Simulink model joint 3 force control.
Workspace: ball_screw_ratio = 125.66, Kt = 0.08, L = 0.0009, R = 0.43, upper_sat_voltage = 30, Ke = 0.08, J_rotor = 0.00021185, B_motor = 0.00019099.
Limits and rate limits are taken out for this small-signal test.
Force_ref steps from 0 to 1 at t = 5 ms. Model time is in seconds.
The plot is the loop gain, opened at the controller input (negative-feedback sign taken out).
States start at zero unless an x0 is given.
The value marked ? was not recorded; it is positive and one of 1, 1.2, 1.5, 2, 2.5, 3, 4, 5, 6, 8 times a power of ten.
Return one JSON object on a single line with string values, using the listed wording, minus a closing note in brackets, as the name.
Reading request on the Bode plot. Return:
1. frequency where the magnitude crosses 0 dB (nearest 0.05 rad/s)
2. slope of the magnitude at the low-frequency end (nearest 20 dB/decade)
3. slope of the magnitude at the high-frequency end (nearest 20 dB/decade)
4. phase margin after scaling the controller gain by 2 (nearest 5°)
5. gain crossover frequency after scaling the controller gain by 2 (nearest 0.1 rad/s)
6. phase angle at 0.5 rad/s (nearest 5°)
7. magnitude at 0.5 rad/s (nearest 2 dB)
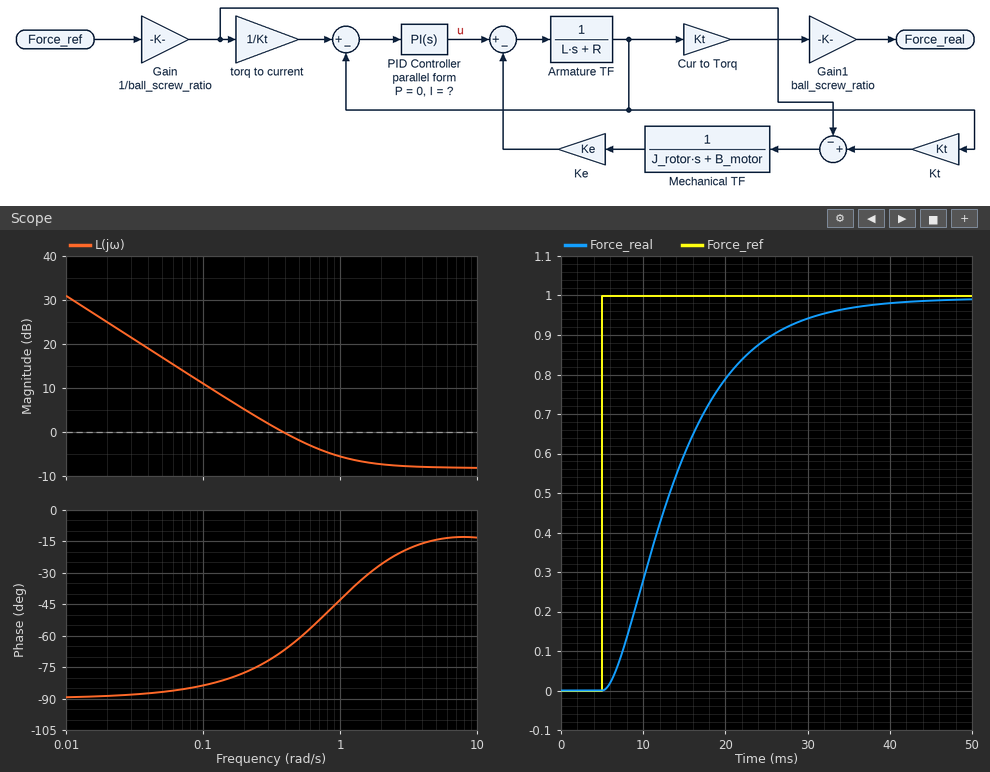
{"frequency where the magnitude crosses 0 dB": "0.40 rad/s", "slope of the magnitude at the low-frequency end": "-20 dB/decade", "slope of the magnitude at the high-frequency end": "0 dB/decade", "phase margin after scaling the controller gain by 2": "140°", "gain crossover frequency after scaling the controller gain by 2": "1.1 rad/s", "phase angle at 0.5 rad/s": "-60°", "magnitude at 0.5 rad/s": "-2 dB"}
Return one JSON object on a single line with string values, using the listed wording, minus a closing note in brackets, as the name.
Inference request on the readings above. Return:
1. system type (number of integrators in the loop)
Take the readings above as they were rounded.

{"system type": "1"}
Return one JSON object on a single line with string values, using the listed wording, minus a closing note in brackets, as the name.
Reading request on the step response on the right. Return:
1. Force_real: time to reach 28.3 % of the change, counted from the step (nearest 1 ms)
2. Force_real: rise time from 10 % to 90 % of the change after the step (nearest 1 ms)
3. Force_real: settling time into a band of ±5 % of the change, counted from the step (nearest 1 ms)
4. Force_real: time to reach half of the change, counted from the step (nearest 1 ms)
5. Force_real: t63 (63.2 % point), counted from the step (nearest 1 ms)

{"Force_real: time to reach 28.3 % of the change, counted from the step": "5 ms", "Force_real: rise time from 10 % to 90 % of the change after the step": "18 ms", "Force_real: settling time into a band of ±5 % of the change, counted from the step": "25 ms", "Force_real: time to reach half of the change, counted from the step": "8 ms", "Force_real: t63 (63.2 % point), counted from the step": "11 ms"}
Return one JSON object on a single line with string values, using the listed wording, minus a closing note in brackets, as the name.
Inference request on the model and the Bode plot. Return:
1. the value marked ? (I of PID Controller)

{"the value marked ?": "12"}
